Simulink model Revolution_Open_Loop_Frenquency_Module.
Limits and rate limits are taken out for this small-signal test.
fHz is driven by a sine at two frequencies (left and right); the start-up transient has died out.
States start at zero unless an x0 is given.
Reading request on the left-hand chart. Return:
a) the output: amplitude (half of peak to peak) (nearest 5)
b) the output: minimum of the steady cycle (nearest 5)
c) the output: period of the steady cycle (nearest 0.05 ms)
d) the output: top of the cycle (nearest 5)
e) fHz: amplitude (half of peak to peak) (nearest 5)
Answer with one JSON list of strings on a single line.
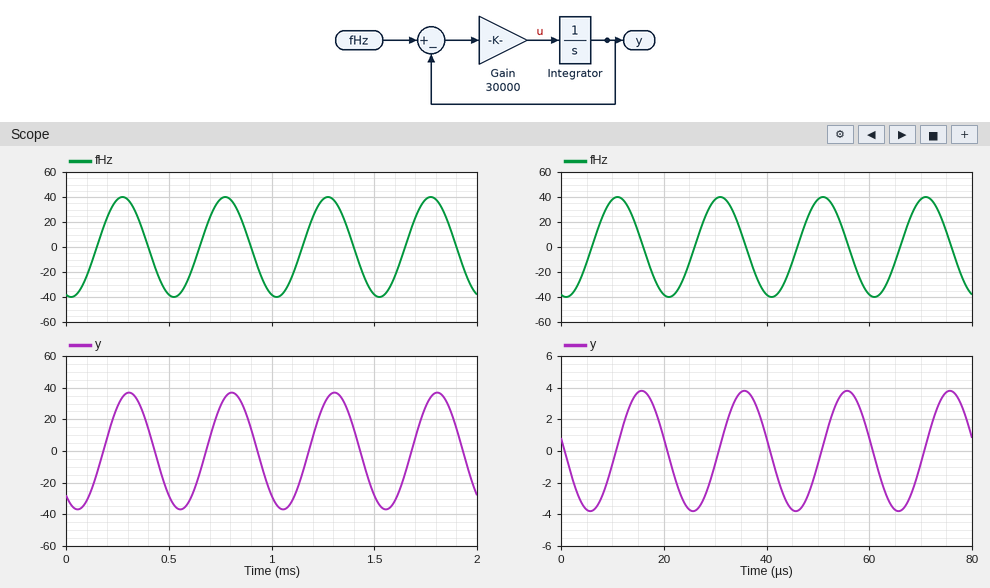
["35", "-35", "0.50 ms", "35", "40"]
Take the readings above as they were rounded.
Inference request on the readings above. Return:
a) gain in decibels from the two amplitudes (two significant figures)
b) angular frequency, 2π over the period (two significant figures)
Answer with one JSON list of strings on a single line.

["-1.2 dB", "13 rad/ms"]
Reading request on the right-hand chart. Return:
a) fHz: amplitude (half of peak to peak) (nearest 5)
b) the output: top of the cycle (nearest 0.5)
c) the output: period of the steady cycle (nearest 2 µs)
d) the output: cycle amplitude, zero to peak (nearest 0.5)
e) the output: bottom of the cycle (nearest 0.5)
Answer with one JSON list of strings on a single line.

["40", "4.0", "20 µs", "4.0", "-4.0"]
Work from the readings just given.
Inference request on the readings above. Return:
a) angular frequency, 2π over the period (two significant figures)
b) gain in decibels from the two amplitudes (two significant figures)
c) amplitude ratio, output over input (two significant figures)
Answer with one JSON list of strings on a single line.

["0.31 rad/µs", "-20 dB", "0.10"]
